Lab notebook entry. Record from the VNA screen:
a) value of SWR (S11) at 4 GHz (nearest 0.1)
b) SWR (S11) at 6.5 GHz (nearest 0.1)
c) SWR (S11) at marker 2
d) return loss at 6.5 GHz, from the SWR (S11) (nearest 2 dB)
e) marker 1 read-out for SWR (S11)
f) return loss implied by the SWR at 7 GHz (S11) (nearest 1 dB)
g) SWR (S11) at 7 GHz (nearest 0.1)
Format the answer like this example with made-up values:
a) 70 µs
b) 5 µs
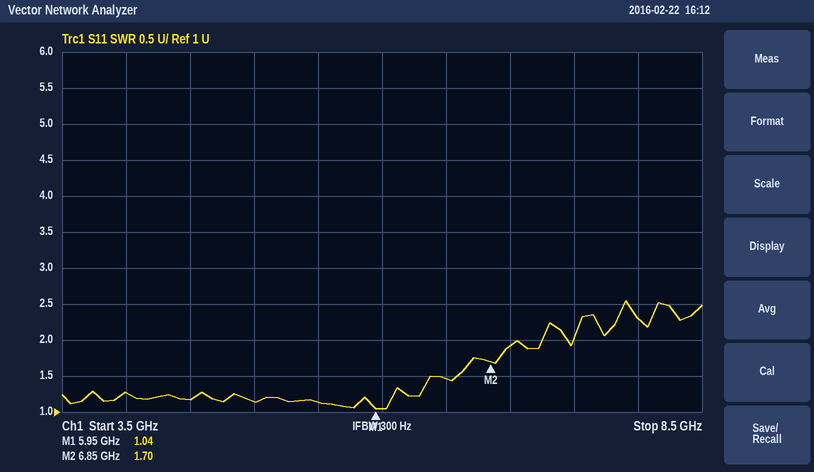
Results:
a) 1.3
b) 1.5
c) 1.70
d) 14 dB
e) 1.04
f) 10 dB
g) 1.9
